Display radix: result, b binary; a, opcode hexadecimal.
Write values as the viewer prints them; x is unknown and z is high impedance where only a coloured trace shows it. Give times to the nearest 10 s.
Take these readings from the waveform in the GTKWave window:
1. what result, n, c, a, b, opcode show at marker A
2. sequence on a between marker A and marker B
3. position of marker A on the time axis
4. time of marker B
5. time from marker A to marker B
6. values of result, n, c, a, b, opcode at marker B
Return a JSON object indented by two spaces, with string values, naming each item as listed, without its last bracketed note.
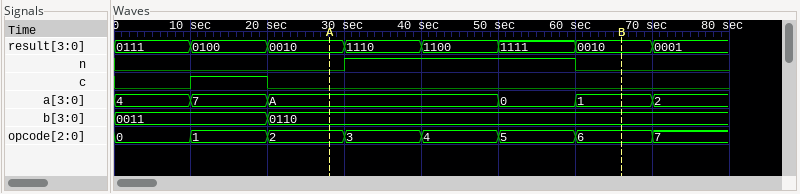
{
  "what result, n, c, a, b, opcode show at marker A": "result=0010, n=0, c=0, a=A, b=0110, opcode=2",
  "sequence on a between marker A and marker B": "A, 0, 1",
  "position of marker A on the time axis": "30 s",
  "time of marker B": "70 s",
  "time from marker A to marker B": "40 s",
  "values of result, n, c, a, b, opcode at marker B": "result=0010, n=0, c=0, a=1, b=0110, opcode=6"
}
